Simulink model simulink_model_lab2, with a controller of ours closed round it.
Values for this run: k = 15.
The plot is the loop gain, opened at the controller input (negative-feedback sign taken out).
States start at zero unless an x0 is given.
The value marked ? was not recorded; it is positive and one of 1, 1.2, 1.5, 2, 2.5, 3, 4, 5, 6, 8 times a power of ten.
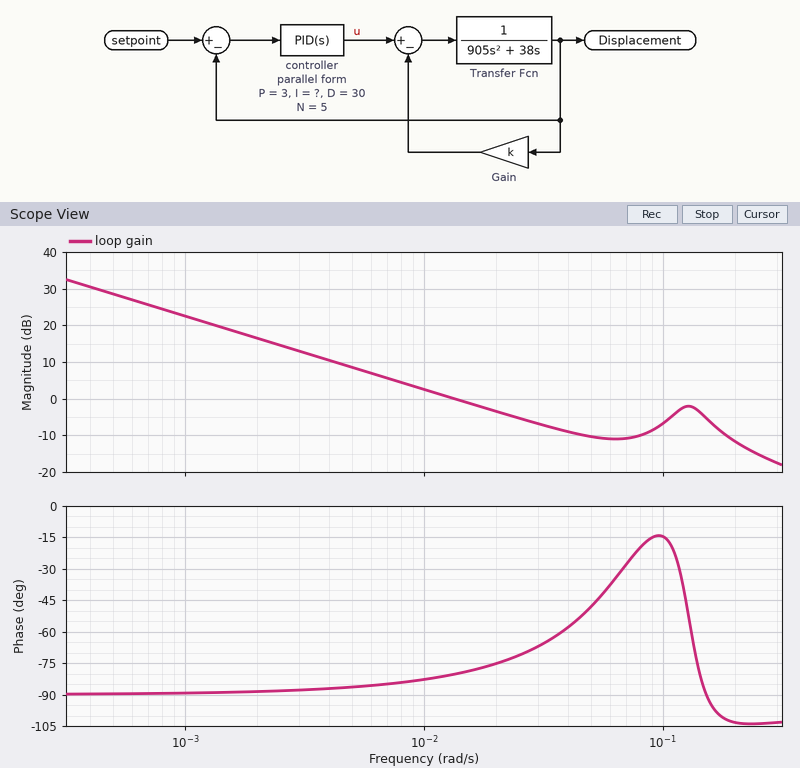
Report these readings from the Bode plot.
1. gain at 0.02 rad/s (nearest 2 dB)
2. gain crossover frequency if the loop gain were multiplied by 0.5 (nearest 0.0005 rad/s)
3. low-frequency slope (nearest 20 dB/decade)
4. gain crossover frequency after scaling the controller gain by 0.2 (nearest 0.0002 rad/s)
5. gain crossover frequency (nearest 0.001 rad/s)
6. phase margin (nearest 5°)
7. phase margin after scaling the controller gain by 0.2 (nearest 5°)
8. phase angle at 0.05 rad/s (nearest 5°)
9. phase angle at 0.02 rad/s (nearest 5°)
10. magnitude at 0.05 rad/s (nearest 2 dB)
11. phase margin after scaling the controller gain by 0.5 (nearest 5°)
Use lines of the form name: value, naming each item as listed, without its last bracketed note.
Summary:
gain at 0.02 rad/s: -4 dB
gain crossover frequency if the loop gain were multiplied by 0.5: 0.0065 rad/s
low-frequency slope: -20 dB/decade
gain crossover frequency after scaling the controller gain by 0.2: 0.0026 rad/s
gain crossover frequency: 0.013 rad/s
phase margin: 100°
phase margin after scaling the controller gain by 0.2: 90°
phase angle at 0.05 rad/s: -50°
phase angle at 0.02 rad/s: -75°
magnitude at 0.05 rad/s: -10 dB
phase margin after scaling the controller gain by 0.5: 95°
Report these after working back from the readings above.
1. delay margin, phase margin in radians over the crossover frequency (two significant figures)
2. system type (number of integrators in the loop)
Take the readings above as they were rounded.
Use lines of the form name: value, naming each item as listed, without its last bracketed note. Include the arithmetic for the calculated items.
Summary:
delay margin, phase margin in radians over the crossover frequency: 100 × π / 180 / 0.013 = 130 s
system type: 1
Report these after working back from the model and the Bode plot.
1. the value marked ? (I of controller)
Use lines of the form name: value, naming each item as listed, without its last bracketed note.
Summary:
the value marked ?: 0.2
